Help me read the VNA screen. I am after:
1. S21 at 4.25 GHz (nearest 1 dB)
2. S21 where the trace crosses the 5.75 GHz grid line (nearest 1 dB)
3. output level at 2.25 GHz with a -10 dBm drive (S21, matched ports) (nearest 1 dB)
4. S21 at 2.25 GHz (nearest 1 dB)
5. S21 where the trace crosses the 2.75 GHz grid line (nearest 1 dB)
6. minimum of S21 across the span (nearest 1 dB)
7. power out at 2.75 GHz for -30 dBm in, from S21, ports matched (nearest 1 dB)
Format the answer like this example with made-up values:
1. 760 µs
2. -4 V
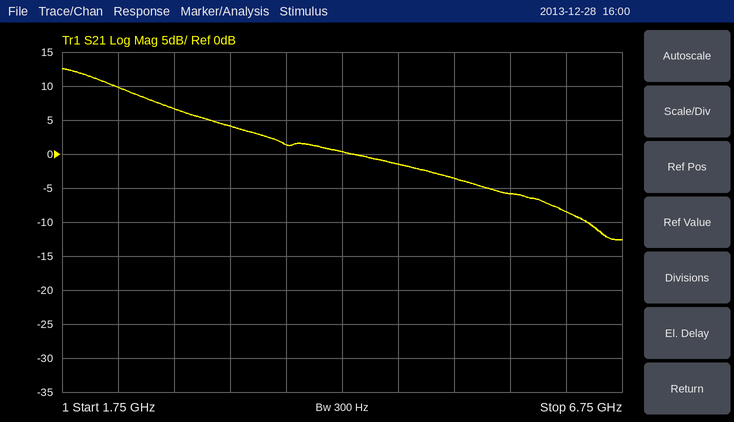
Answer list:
1. 0 dB
2. -6 dB
3. 0 dBm
4. 10 dB
5. 7 dB
6. -13 dB
7. -23 dBm
